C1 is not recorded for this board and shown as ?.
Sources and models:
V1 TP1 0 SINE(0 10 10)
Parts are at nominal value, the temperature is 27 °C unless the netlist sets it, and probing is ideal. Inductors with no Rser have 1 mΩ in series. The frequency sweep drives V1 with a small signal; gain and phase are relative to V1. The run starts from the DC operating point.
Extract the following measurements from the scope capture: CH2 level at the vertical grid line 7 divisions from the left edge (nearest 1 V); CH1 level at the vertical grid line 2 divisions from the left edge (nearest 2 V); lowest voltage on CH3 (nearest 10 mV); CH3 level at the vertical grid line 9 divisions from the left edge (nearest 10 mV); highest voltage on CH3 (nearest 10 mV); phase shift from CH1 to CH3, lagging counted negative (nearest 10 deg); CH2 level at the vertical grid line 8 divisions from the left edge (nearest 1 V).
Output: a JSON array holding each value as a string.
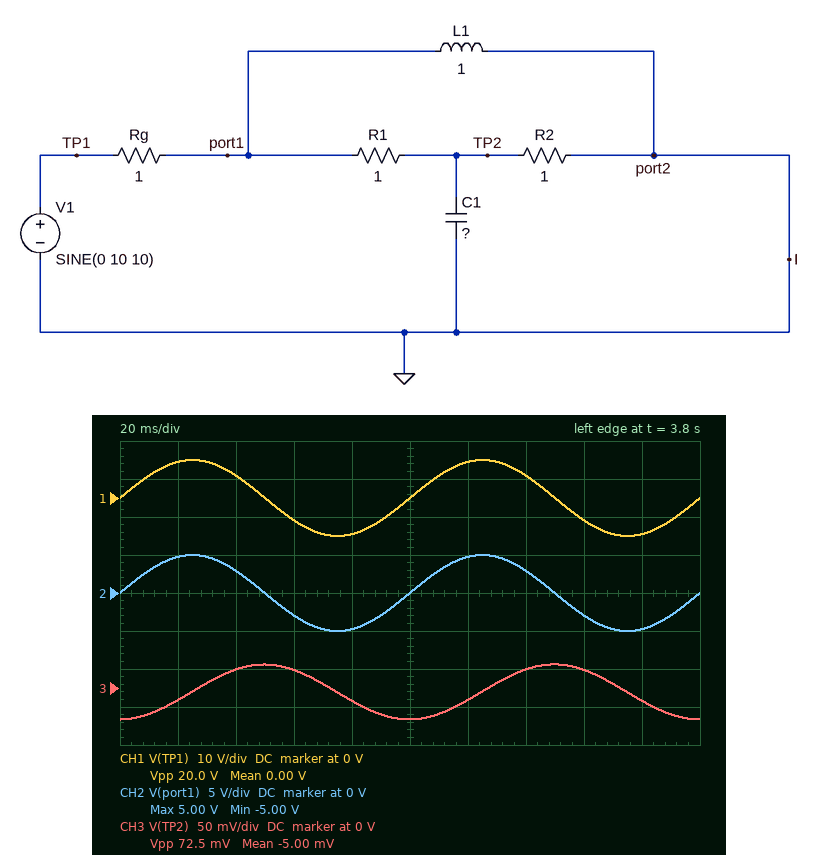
["3 V", "6 V", "-40 mV", "-20 mV", "30 mV", "-90 deg", "-3 V"]
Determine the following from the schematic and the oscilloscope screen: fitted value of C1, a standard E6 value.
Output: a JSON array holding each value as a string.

["2.2 F"]
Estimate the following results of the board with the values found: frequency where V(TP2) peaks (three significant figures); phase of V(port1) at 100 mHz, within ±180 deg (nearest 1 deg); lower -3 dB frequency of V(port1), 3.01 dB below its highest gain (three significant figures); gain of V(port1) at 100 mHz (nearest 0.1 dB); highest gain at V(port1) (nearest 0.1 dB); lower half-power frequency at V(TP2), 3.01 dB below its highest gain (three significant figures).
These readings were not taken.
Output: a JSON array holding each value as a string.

["107 mHz", "39 deg", "67.0 mHz", "-6.6 dB", "-5.6 dB", "48.7 mHz"]
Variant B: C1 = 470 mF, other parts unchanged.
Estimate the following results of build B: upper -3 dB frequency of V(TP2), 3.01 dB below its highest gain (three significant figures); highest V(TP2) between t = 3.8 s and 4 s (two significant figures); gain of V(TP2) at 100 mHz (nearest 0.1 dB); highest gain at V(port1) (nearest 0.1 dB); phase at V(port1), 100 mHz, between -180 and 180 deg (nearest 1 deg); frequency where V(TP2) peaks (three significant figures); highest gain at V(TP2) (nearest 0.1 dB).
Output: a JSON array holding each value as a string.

["668 mHz", "170 mV", "-12.7 dB", "-4.2 dB", "45 deg", "232 mHz", "-10.8 dB"]
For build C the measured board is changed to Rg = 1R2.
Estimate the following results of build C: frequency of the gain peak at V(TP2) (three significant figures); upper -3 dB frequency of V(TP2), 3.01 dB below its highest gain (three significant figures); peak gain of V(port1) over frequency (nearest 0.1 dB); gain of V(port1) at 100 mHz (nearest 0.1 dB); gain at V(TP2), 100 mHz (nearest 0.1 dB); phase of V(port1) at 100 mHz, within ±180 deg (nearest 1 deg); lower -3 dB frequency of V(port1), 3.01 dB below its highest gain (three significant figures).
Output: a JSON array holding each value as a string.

["112 mHz", "244 mHz", "-6.5 dB", "-7.7 dB", "-15.4 dB", "42 deg", "71.7 mHz"]
